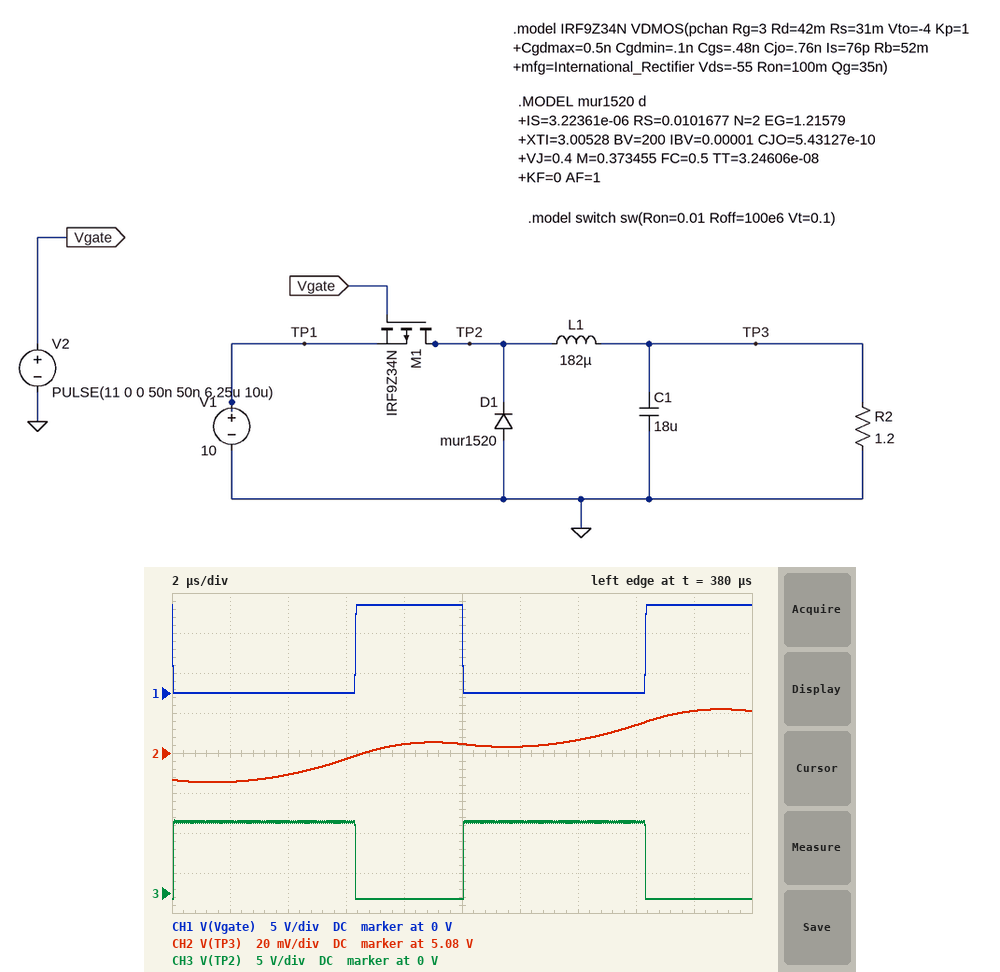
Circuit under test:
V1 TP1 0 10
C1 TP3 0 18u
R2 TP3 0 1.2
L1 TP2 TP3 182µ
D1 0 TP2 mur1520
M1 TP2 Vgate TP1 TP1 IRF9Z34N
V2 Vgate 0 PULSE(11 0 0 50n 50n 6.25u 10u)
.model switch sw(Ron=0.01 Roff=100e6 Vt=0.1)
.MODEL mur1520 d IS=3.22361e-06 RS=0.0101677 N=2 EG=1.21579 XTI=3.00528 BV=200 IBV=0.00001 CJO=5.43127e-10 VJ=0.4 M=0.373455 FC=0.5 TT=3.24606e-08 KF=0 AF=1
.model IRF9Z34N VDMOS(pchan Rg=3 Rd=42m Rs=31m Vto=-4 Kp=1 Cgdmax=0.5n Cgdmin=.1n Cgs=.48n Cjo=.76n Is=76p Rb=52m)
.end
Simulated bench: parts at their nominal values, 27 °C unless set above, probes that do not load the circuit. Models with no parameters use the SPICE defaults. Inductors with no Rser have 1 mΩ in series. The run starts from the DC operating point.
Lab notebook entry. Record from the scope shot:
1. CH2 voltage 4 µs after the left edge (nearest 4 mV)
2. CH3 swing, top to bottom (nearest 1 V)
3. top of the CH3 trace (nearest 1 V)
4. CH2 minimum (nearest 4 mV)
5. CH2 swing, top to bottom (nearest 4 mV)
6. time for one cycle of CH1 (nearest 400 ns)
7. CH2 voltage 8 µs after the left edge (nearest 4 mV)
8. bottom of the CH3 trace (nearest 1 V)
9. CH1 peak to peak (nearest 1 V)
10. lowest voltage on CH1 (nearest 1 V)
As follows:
5.068 V
10 V
9 V
5.064 V
36 mV
10.0 µs
5.084 V
-1 V
11 V
0 V
